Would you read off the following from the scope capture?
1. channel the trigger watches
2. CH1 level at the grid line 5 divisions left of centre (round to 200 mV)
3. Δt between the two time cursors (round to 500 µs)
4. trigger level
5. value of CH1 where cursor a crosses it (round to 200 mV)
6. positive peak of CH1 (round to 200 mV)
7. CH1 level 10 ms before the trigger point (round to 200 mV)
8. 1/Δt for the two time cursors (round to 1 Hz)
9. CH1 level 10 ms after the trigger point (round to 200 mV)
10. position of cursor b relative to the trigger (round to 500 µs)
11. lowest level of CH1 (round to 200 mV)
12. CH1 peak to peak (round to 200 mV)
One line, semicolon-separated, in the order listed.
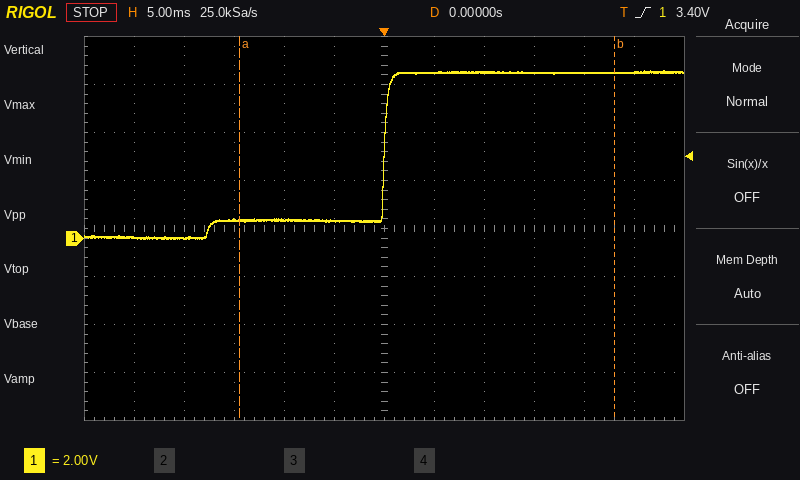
CH1; 0.0 V; 37.5 ms; 3.40 V; 800 mV; 7.0 V; 800 mV; 27 Hz; 7.0 V; +23.0 ms; 0.0 V; 7.0 V
